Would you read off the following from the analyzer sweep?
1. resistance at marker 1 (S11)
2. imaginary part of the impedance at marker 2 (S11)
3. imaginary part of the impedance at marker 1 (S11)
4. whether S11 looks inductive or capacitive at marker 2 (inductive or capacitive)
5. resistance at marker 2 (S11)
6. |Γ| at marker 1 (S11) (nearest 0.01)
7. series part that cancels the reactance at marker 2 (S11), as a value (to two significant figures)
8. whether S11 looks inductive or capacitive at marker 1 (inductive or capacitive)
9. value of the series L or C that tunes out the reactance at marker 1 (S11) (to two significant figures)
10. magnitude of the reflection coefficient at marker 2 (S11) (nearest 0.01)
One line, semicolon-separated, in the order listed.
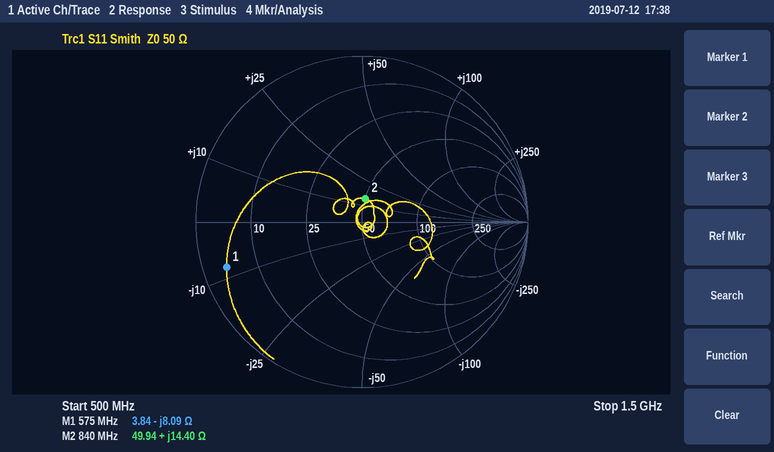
3.84 Ω; +14.40 Ω; -8.09 Ω; inductive; 49.94 Ω; 0.86; 13 pF; capacitive; 2.2 nH; 0.14
